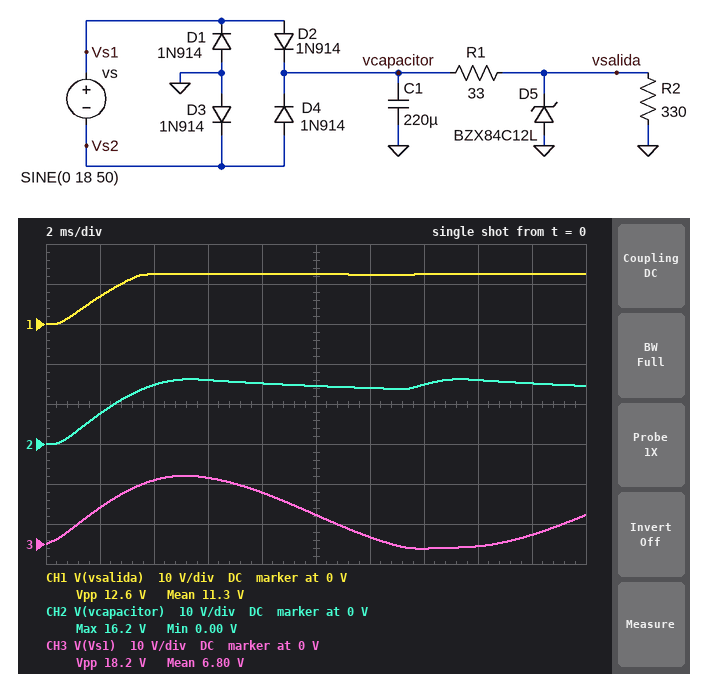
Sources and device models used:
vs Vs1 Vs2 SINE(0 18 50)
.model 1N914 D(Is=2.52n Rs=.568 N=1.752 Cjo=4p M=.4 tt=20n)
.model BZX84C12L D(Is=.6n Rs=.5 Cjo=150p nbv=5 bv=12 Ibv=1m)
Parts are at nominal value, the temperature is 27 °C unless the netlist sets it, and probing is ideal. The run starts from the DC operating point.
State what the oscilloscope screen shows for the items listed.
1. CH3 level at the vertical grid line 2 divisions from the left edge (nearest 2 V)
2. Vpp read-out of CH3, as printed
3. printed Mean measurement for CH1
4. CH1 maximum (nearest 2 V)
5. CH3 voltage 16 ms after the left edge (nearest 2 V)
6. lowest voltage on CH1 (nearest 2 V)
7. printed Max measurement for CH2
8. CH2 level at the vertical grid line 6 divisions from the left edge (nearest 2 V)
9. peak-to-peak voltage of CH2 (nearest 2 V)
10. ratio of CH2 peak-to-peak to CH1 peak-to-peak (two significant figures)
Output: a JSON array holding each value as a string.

["16 V", "18.2 V", "11.3 V", "12 V", "0 V", "0 V", "16.2 V", "14 V", "16 V", "1.3"]
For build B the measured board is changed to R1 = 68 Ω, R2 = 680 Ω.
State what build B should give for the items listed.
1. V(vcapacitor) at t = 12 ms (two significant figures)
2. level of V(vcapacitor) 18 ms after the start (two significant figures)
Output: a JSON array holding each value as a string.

["15 V", "16 V"]
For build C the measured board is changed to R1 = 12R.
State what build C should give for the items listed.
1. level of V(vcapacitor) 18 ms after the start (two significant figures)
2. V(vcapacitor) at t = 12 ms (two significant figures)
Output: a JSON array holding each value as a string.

["14 V", "13 V"]
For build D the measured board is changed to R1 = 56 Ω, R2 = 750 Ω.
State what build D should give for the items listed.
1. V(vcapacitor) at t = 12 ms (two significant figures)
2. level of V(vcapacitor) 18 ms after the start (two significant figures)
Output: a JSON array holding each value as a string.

["15 V", "16 V"]
